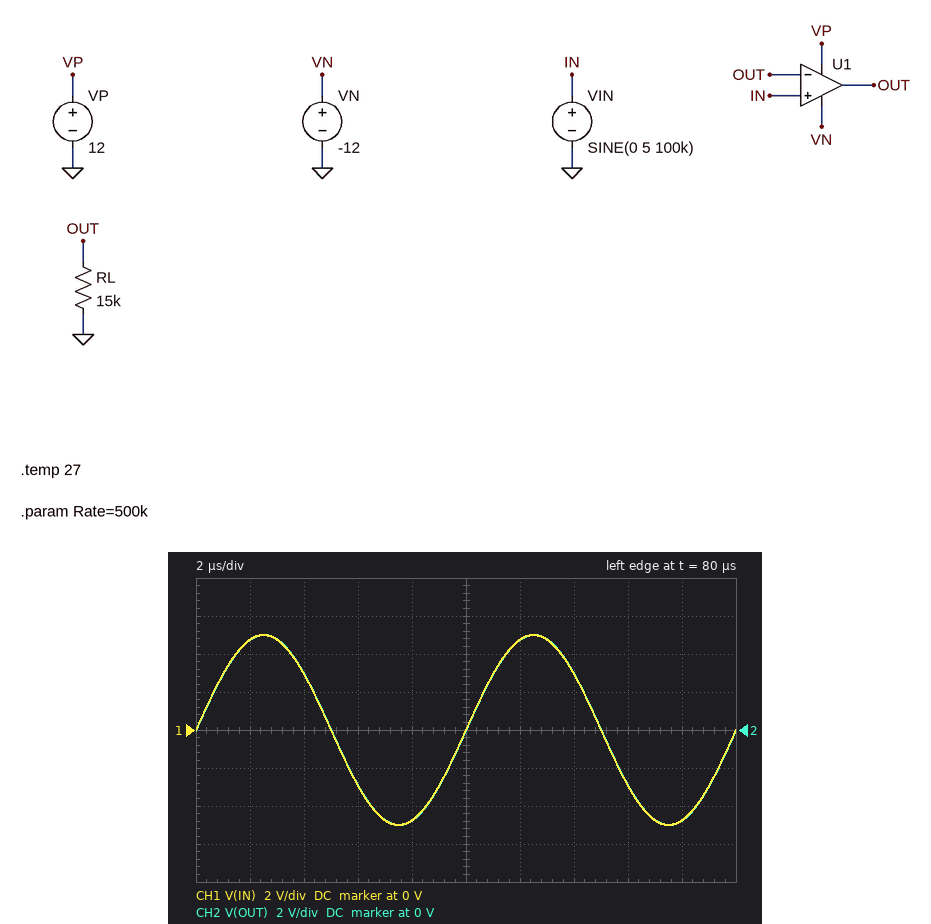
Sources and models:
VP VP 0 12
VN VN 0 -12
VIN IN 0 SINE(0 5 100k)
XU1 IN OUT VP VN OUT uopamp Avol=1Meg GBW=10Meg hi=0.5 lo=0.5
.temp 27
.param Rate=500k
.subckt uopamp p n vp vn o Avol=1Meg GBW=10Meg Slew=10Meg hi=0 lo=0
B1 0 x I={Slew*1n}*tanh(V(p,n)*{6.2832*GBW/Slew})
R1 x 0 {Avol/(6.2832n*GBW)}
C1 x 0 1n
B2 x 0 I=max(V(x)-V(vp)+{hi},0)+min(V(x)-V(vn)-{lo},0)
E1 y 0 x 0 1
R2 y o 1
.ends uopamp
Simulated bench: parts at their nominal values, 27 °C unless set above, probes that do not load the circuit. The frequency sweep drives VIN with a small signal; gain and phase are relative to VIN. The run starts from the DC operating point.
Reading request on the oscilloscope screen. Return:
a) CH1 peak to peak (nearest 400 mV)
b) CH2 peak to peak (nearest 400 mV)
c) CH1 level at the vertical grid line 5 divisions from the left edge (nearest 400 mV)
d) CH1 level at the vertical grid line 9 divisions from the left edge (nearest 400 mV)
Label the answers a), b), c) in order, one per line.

a) 10.0 V
b) 10.0 V
c) 0 V
d) -4.8 V
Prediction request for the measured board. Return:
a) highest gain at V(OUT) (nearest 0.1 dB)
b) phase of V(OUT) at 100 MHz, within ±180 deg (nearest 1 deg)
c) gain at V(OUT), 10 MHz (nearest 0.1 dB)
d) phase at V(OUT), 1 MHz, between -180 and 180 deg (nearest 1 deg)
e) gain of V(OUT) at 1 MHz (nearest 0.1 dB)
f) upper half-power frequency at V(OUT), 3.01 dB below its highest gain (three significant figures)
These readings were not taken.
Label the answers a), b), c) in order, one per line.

a) 0 dB
b) -84 deg
c) -3.0 dB
d) -6 deg
e) 0 dB
f) 10.0 MHz
